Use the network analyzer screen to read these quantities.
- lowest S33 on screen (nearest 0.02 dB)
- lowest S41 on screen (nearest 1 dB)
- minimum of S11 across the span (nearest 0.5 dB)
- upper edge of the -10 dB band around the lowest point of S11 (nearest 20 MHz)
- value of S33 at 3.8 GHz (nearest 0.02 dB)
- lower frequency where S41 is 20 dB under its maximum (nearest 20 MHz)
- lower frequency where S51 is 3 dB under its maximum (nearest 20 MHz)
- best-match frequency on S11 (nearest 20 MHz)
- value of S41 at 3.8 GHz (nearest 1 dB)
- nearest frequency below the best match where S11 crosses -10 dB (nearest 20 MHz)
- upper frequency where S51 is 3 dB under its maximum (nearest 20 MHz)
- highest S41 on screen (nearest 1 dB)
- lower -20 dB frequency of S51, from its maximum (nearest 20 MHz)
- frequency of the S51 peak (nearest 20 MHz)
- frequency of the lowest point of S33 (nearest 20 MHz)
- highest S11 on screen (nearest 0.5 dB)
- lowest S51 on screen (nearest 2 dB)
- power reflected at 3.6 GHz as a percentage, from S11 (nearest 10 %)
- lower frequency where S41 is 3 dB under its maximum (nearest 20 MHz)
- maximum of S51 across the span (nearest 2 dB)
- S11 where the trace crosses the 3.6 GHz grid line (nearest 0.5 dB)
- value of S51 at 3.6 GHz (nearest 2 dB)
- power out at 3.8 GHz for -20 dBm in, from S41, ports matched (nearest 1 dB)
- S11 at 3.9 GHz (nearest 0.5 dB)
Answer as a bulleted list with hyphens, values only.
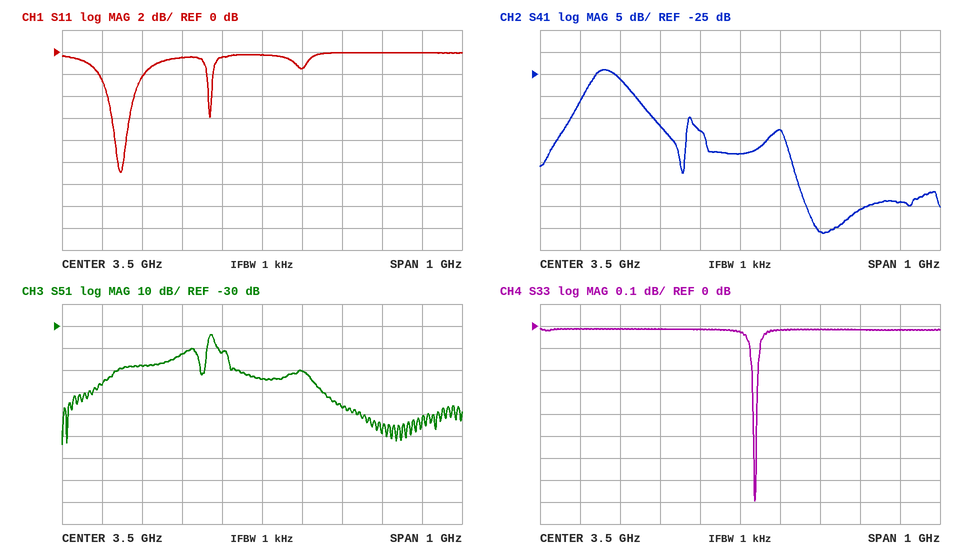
- -0.80 dB
- -61 dB
- -11.0 dB
- 3.16 GHz
- -0.02 dB
- 3.02 GHz
- 3.36 GHz
- 3.14 GHz
- -56 dB
- 3.14 GHz
- 3.38 GHz
- -24 dB
- 3.12 GHz
- 3.38 GHz
- 3.54 GHz
- 0.0 dB
- -84 dB
- 70 %
- 3.12 GHz
- -34 dB
- -1.5 dB
- -50 dB
- -76 dBm
- 0.0 dB
